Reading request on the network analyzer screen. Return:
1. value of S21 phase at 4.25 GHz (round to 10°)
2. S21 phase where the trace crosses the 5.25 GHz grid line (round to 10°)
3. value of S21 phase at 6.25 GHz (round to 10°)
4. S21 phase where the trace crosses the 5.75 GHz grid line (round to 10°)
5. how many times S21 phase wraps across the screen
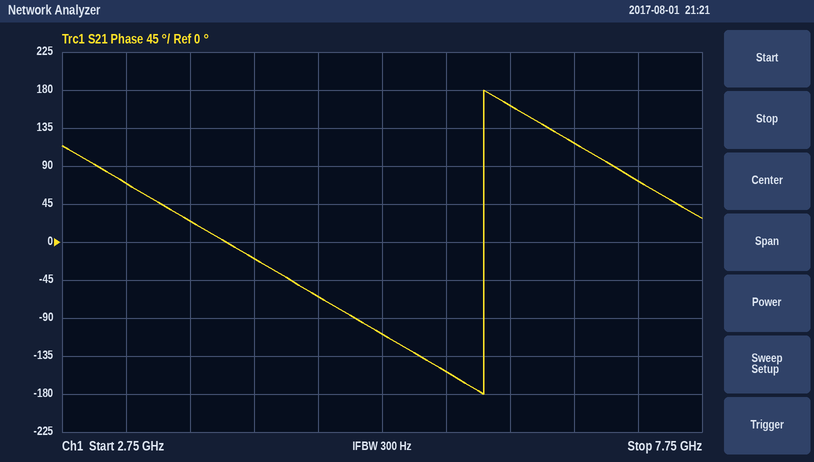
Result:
-20°
-110°
160°
-150°
1
